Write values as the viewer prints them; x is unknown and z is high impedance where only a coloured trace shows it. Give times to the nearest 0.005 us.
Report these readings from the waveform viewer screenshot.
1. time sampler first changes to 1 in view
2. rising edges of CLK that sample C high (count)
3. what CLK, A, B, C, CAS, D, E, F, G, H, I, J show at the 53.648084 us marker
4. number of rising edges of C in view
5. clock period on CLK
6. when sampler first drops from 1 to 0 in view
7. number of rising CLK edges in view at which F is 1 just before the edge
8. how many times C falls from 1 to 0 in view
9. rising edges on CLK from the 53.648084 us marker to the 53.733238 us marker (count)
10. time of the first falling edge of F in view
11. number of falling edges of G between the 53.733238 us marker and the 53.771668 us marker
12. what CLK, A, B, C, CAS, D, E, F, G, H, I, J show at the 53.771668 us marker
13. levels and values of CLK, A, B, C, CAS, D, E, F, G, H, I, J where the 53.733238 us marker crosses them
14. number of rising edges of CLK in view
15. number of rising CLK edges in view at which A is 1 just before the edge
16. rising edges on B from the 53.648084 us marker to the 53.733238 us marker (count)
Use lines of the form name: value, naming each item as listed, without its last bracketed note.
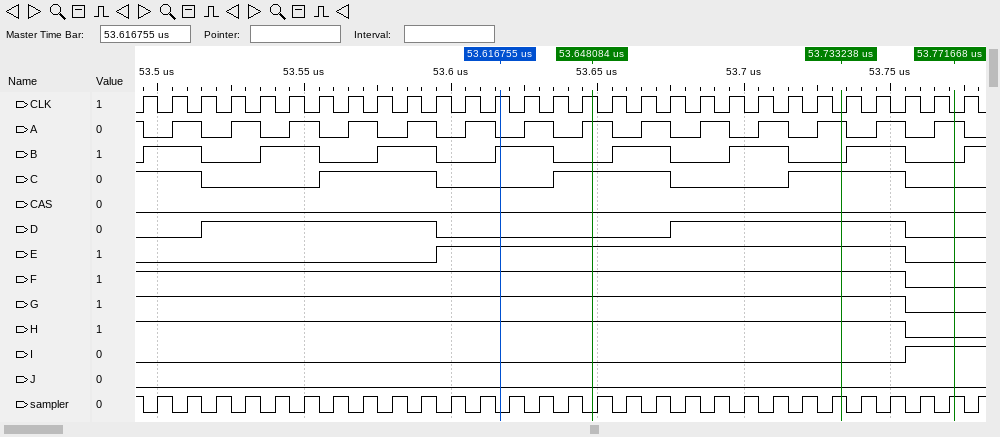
time sampler first changes to 1 in view: 53.5 us
rising edges of CLK that sample C high: 15
what CLK, A, B, C, CAS, D, E, F, G, H, I, J show at the 53.648084 us marker: CLK=1, A=1, B=0, C=1, CAS=0, D=0, E=1, F=1, G=1, H=1, I=0, J=0
number of rising edges of C in view: 3
clock period on CLK: 0.01 us
when sampler first drops from 1 to 0 in view: 53.495 us
number of rising CLK edges in view at which F is 1 just before the edge: 27
how many times C falls from 1 to 0 in view: 4
rising edges on CLK from the 53.648084 us marker to the 53.733238 us marker: 8
time of the first falling edge of F in view: 53.755 us
number of falling edges of G between the 53.733238 us marker and the 53.771668 us marker: 1
what CLK, A, B, C, CAS, D, E, F, G, H, I, J show at the 53.771668 us marker: CLK=0, A=1, B=0, C=0, CAS=0, D=0, E=0, F=0, G=0, H=0, I=1, J=0
levels and values of CLK, A, B, C, CAS, D, E, F, G, H, I, J where the 53.733238 us marker crosses them: CLK=0, A=1, B=0, C=1, CAS=0, D=1, E=1, F=1, G=1, H=1, I=0, J=0
number of rising edges of CLK in view: 29
number of rising CLK edges in view at which A is 1 just before the edge: 15
rising edges on B from the 53.648084 us marker to the 53.733238 us marker: 2
